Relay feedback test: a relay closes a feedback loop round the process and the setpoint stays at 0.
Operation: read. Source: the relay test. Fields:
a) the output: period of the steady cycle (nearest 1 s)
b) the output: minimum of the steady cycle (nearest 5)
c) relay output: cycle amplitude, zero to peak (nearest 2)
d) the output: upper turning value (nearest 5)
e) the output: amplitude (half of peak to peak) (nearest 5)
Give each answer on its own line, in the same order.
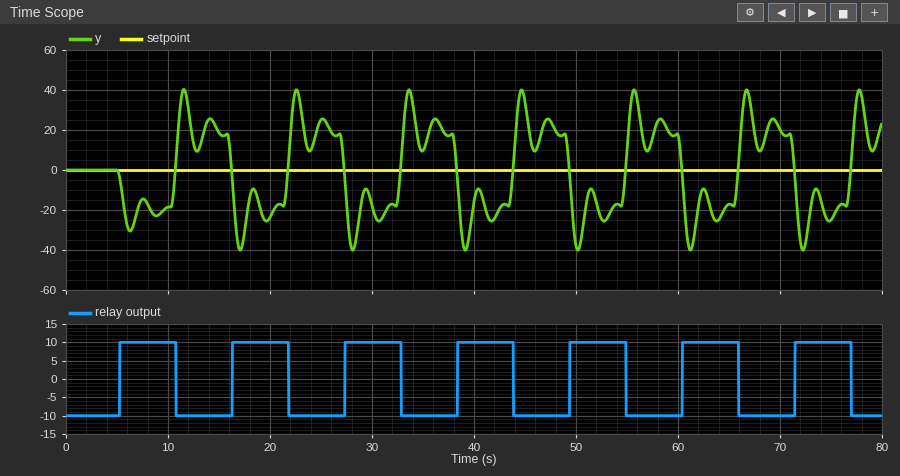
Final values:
11 s
-40
10
40
40
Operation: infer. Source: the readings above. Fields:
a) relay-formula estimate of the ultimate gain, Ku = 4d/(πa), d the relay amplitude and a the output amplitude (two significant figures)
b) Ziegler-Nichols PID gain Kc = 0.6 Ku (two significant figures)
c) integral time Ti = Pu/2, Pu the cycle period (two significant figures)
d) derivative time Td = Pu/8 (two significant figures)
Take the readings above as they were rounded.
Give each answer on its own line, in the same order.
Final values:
0.32
0.19
5.5 s
1.4 s
